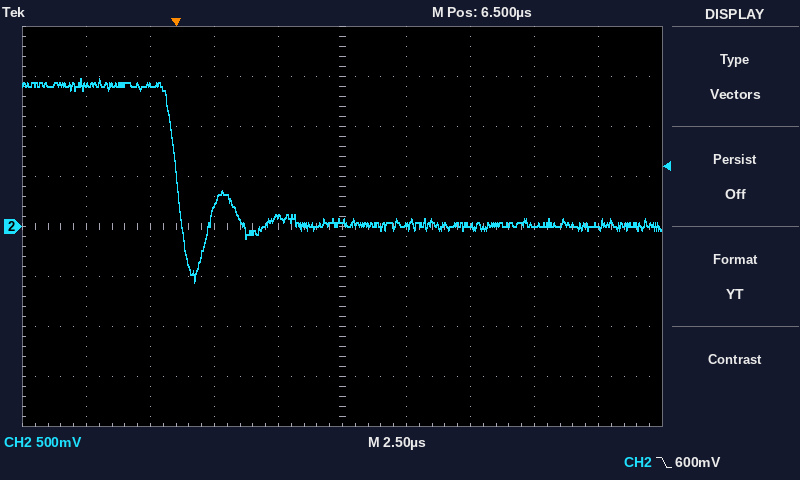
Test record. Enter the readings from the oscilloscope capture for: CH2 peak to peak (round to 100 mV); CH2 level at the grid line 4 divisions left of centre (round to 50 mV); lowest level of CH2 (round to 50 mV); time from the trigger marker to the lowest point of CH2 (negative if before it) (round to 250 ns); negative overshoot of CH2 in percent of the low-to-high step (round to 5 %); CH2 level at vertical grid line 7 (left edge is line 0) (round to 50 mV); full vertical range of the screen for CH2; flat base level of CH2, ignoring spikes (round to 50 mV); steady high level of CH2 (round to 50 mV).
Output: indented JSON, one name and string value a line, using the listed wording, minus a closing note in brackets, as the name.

{
  "CH2 peak to peak": "2.00 V",
  "CH2 level at the grid line 4 divisions left of centre": "1.40 V",
  "lowest level of CH2": "-550 mV",
  "time from the trigger marker to the lowest point of CH2 (negative if before it)": "+750 ns",
  "negative overshoot of CH2 in percent of the low-to-high step": "40 %",
  "CH2 level at vertical grid line 7 (left edge is line 0)": "0 mV",
  "full vertical range of the screen for CH2": "4 V",
  "flat base level of CH2, ignoring spikes": "0 mV",
  "steady high level of CH2": "1.40 V"
}
